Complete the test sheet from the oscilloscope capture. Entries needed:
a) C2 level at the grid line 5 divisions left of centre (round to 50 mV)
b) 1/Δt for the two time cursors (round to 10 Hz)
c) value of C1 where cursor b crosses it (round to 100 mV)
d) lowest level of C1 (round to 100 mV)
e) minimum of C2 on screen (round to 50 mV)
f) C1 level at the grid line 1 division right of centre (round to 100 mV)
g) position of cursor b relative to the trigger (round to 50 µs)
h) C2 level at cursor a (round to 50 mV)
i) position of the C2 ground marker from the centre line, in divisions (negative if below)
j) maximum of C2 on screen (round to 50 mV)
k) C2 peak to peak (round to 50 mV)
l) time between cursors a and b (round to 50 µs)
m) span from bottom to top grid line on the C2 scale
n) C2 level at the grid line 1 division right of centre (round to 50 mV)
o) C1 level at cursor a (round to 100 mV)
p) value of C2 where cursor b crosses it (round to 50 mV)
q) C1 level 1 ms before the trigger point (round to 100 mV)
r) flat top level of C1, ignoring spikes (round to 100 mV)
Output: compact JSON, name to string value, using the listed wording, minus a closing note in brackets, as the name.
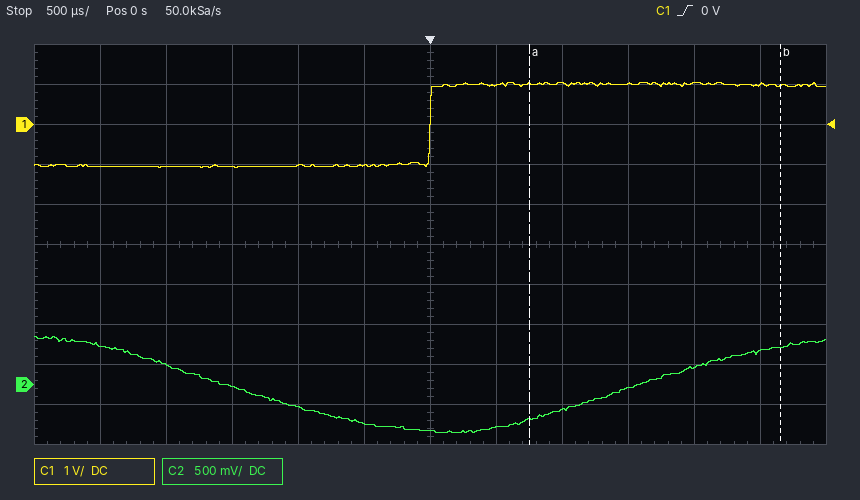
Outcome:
{"C2 level at the grid line 5 divisions left of centre": "500 mV", "1/Δt for the two time cursors": "530 Hz", "value of C1 where cursor b crosses it": "1.0 V", "lowest level of C1": "-1.1 V", "minimum of C2 on screen": "-600 mV", "C1 level at the grid line 1 division right of centre": "1.0 V", "position of cursor b relative to the trigger": "+2.65 ms", "C2 level at cursor a": "-450 mV", "position of the C2 ground marker from the centre line, in divisions": "-3.5 div", "maximum of C2 on screen": "600 mV", "C2 peak to peak": "1.20 V", "time between cursors a and b": "1.90 ms", "span from bottom to top grid line on the C2 scale": "5 V", "C2 level at the grid line 1 division right of centre": "-550 mV", "C1 level at cursor a": "1.0 V", "value of C2 where cursor b crosses it": "450 mV", "C1 level 1 ms before the trigger point": "-1.0 V", "flat top level of C1, ignoring spikes": "1.0 V"}
